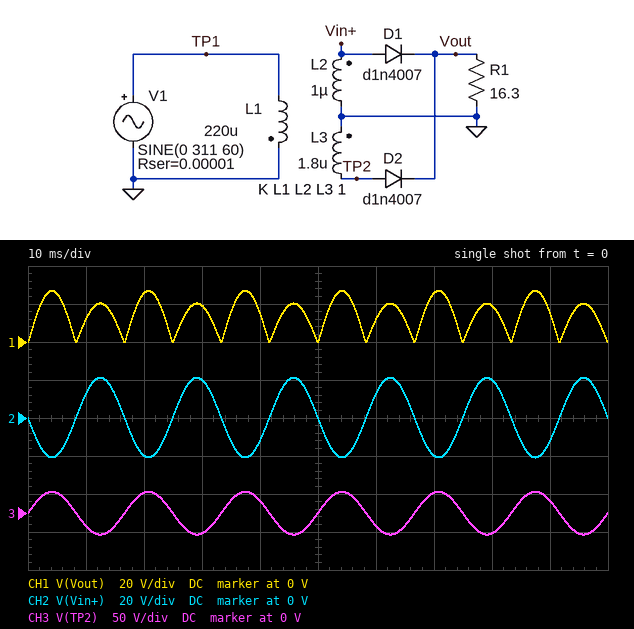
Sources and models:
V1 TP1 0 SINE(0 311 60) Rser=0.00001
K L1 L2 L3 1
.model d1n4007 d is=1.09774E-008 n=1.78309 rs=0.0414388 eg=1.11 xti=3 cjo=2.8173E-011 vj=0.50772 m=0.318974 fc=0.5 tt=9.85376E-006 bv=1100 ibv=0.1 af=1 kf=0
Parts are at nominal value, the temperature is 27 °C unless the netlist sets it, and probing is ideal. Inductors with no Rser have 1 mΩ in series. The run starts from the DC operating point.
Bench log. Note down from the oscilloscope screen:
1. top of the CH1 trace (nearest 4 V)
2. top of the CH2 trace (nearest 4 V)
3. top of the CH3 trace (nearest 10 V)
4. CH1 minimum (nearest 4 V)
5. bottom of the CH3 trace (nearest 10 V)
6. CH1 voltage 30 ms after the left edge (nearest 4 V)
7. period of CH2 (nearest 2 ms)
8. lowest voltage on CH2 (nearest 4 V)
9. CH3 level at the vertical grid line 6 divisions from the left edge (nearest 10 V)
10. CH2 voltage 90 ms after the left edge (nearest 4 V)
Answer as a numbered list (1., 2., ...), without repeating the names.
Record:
1. 28 V
2. 20 V
3. 30 V
4. 0 V
5. -30 V
6. 20 V
7. 16 ms
8. -20 V
9. -20 V
10. -12 V
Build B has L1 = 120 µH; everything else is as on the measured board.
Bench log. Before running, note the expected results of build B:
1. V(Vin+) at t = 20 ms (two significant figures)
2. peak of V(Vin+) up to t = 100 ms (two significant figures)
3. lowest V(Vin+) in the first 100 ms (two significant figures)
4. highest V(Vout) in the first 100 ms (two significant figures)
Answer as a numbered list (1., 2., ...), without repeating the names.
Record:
1. -27 V
2. 29 V
3. -28 V
4. 37 V
